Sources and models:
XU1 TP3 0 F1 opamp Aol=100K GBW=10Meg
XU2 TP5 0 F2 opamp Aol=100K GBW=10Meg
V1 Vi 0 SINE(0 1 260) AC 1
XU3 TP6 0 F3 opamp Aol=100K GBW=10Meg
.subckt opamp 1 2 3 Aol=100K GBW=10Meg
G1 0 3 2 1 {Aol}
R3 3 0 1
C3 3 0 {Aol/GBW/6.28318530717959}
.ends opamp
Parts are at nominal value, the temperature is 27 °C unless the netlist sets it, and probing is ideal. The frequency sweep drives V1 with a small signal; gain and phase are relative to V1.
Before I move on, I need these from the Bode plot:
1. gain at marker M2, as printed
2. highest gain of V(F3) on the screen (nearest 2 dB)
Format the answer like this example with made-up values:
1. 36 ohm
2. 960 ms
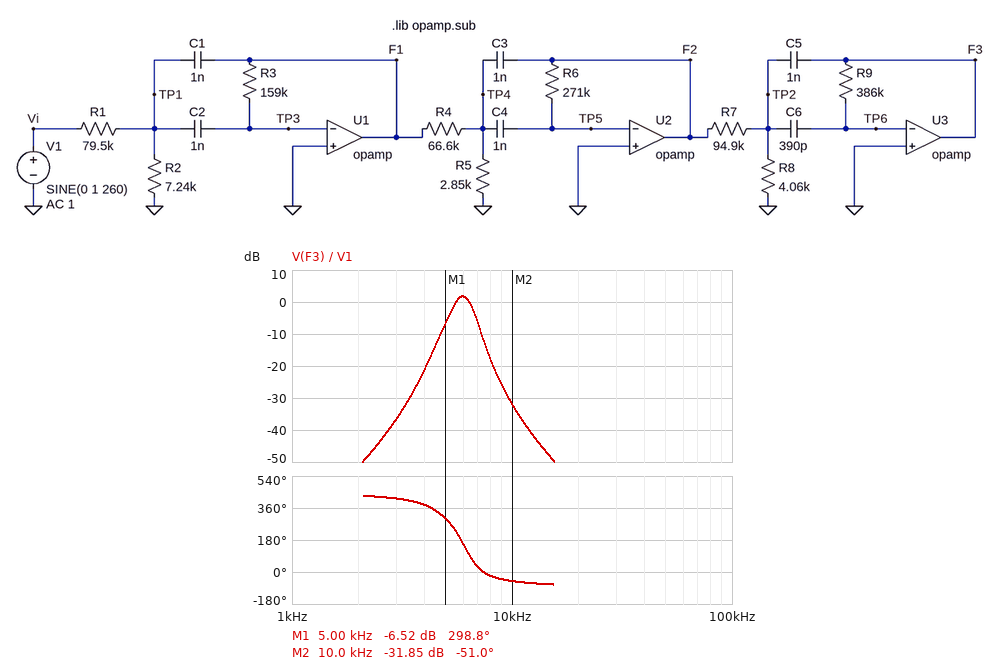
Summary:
1. -31.85 dB
2. 2 dB
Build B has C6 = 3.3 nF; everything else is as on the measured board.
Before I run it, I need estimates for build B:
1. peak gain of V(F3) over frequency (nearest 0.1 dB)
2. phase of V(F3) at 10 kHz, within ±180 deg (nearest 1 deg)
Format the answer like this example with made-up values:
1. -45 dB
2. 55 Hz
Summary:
1. -5.1 dB
2. -62 deg
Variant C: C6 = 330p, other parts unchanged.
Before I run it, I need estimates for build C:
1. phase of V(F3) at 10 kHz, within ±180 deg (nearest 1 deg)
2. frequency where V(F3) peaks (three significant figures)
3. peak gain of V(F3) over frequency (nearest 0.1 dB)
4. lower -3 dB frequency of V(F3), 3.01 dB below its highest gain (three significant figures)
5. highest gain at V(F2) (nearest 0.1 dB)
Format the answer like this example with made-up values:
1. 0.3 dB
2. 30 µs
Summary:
1. -47 deg
2. 5.92 kHz
3. -2.2 dB
4. 5.39 kHz
5. 4.0 dB
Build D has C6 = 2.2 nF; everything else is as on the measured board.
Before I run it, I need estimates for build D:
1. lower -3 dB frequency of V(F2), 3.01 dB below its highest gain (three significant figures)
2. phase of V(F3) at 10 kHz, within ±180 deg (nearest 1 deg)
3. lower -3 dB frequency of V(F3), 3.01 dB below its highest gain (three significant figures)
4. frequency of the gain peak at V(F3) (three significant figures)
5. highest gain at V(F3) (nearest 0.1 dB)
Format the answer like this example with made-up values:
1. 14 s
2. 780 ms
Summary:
1. 5.02 kHz
2. -62 deg
3. 4.66 kHz
4. 5.56 kHz
5. -4.2 dB
